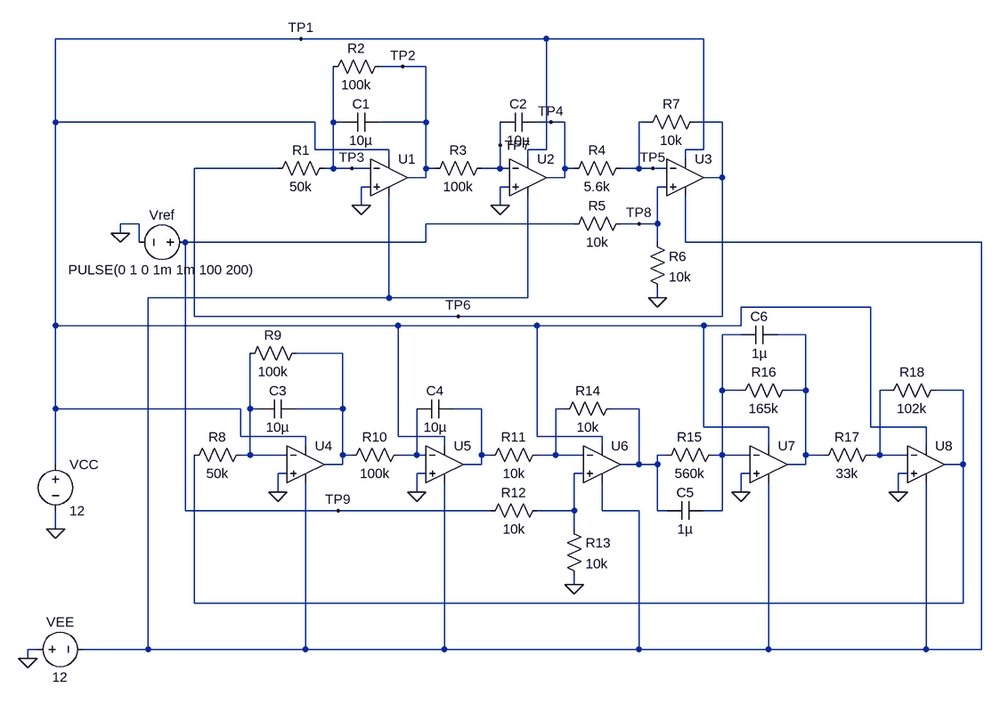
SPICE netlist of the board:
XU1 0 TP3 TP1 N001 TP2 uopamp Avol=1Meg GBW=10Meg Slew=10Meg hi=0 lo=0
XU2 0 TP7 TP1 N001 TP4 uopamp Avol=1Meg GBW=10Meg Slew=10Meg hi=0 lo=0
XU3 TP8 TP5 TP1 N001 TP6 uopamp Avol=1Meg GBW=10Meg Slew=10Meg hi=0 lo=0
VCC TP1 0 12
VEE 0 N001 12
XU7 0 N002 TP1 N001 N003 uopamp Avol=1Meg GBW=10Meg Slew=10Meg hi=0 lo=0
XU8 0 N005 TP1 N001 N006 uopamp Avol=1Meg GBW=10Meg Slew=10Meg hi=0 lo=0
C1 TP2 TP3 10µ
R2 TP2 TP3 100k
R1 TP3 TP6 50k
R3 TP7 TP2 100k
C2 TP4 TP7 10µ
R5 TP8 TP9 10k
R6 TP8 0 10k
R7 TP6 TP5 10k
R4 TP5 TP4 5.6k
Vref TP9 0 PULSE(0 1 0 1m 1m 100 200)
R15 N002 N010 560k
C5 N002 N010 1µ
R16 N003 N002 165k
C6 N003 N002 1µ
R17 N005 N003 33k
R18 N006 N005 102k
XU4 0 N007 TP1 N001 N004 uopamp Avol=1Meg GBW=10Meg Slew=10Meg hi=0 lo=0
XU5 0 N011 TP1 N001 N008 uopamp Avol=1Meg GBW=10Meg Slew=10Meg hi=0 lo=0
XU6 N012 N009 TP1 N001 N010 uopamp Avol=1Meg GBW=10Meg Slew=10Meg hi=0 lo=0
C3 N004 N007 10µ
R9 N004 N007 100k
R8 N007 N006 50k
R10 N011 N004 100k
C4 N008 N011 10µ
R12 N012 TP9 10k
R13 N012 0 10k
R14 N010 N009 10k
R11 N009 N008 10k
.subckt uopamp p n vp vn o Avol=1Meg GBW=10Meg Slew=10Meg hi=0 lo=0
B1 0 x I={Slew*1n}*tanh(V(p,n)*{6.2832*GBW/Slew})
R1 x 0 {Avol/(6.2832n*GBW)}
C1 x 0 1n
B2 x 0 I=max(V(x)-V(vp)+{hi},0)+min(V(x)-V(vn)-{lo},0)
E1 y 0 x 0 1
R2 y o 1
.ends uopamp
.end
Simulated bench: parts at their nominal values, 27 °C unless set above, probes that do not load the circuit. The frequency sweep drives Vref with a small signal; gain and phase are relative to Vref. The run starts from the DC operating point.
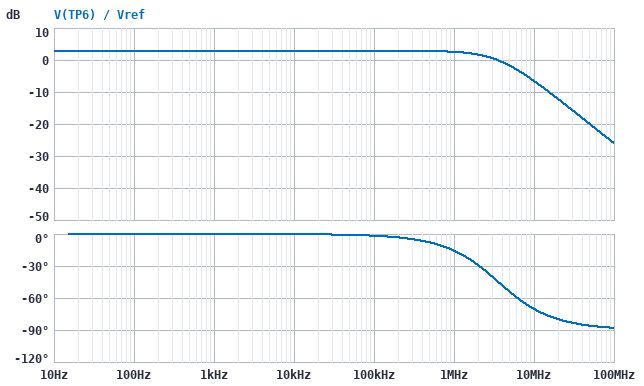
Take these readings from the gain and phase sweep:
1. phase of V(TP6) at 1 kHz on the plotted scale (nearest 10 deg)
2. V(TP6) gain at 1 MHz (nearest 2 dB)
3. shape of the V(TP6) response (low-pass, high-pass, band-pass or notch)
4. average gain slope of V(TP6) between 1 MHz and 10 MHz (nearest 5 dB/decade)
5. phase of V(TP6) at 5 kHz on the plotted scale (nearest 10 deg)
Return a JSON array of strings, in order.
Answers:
["0 deg", "2 dB", "low-pass", "-10 dB/decade", "0 deg"]
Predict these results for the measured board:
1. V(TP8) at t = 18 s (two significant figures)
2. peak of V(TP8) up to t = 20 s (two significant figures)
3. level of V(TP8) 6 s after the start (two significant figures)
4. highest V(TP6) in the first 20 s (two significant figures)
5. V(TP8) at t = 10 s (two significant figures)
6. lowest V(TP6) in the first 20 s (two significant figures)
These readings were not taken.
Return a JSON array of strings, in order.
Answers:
["500 mV", "500 mV", "500 mV", "1.4 V", "500 mV", "-590 mV"]
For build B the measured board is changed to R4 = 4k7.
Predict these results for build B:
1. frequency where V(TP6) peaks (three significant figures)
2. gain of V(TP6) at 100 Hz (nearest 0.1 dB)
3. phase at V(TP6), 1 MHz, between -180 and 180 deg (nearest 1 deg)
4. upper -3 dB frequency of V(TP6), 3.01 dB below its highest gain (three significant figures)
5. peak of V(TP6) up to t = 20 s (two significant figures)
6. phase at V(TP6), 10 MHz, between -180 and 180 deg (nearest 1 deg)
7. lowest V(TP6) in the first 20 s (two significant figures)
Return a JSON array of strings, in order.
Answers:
["345 mHz", "3.9 dB", "-17 deg", "487 mHz", "1.6 V", "-72 deg", "-710 mV"]
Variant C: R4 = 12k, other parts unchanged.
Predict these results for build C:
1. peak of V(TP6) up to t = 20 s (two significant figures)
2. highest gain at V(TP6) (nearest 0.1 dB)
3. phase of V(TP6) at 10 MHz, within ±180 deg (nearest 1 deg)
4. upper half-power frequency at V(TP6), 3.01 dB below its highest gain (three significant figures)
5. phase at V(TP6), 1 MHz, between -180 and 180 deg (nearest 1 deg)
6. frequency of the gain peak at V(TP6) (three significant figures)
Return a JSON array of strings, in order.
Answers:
["920 mV", "3.8 dB", "-61 deg", "483 mHz", "-10 deg", "229 mHz"]
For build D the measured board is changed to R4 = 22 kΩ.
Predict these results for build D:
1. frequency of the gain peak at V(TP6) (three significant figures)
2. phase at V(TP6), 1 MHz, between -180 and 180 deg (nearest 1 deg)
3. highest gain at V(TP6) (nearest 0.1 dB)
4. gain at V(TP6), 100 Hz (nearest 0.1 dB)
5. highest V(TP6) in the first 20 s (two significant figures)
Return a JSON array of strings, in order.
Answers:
["179 mHz", "-8 deg", "0.4 dB", "-2.8 dB", "730 mV"]
